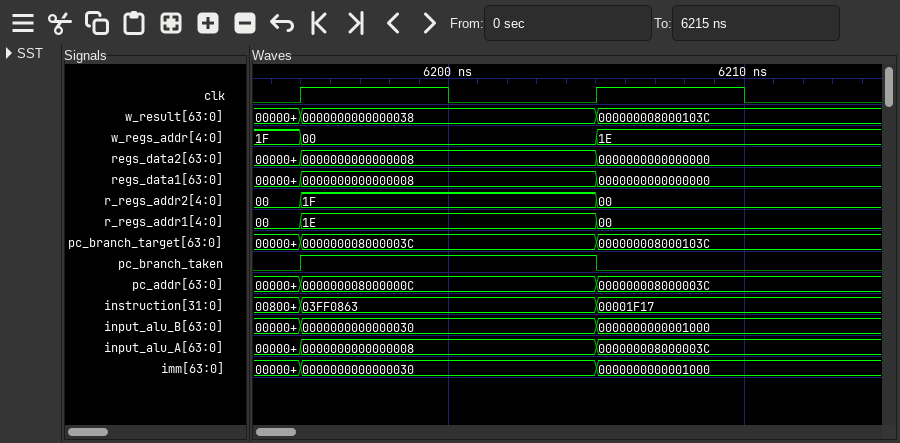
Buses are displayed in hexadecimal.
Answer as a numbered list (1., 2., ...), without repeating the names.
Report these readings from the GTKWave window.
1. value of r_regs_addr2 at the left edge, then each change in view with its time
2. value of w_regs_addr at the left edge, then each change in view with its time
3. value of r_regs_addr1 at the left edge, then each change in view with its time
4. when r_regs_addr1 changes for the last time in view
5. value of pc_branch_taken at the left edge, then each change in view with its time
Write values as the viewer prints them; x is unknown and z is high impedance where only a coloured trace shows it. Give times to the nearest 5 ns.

1. 00, 1F at 6195 ns, 00 at 6205 ns
2. 1F, 00 at 6195 ns, 1E at 6205 ns
3. 00, 1E at 6195 ns, 00 at 6205 ns
4. 6205 ns
5. 0, 1 at 6195 ns, 0 at 6205 ns
